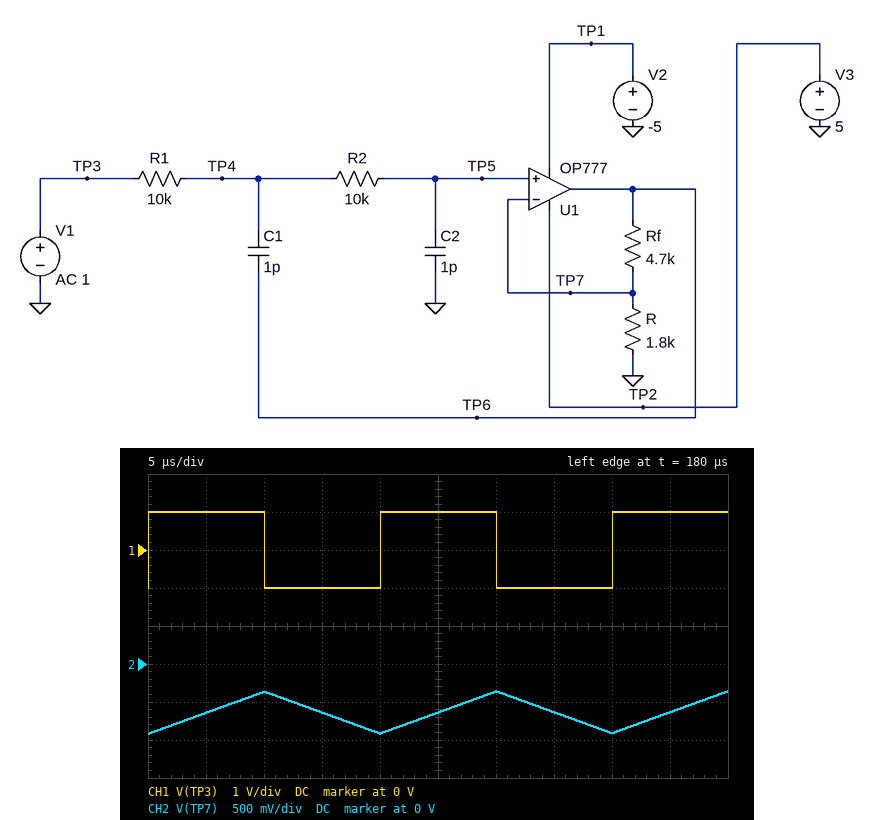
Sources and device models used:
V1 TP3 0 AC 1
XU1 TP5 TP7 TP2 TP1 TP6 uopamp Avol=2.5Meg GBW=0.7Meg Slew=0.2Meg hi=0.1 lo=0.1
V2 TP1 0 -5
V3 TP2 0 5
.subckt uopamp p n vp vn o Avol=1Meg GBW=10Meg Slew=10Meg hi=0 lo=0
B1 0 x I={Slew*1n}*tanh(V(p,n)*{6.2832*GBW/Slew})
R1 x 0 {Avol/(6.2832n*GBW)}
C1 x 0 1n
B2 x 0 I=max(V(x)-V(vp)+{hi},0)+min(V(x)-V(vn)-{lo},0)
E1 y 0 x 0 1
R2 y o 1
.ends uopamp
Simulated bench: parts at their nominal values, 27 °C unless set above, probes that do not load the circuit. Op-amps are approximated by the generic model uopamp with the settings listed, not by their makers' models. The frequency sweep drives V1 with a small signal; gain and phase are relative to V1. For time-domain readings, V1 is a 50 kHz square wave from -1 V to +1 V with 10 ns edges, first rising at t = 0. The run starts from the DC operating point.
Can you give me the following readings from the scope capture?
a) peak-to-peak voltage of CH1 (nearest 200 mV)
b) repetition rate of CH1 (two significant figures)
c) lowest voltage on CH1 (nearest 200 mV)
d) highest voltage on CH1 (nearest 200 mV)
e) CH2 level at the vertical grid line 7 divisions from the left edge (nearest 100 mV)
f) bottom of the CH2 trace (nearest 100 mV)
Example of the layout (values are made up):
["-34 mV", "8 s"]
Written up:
["2.0 V", "50 kHz", "-1.0 V", "1.0 V", "-600 mV", "-900 mV"]
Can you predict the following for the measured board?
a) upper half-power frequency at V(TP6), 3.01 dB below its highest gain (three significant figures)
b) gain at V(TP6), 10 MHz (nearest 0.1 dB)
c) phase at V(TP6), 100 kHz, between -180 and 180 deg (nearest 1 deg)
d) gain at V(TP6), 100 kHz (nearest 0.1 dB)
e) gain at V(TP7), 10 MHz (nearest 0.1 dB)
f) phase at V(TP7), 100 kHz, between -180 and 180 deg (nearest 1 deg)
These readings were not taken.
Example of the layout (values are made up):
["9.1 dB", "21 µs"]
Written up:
["203 kHz", "-29.0 dB", "-27 deg", "10.2 dB", "-40.1 dB", "-27 deg"]
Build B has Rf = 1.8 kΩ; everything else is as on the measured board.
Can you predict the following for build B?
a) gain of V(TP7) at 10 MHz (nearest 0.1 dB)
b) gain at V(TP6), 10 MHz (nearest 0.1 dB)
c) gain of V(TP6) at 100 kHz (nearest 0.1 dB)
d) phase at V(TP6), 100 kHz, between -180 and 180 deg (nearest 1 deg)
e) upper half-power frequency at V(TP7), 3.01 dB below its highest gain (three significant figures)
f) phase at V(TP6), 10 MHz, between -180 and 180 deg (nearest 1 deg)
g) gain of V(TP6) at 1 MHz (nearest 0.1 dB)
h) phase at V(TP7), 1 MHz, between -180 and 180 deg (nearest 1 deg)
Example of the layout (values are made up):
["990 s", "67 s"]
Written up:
["-35.0 dB", "-29.0 dB", "5.7 dB", "-16 deg", "366 kHz", "-161 deg", "-3.4 dB", "-81 deg"]
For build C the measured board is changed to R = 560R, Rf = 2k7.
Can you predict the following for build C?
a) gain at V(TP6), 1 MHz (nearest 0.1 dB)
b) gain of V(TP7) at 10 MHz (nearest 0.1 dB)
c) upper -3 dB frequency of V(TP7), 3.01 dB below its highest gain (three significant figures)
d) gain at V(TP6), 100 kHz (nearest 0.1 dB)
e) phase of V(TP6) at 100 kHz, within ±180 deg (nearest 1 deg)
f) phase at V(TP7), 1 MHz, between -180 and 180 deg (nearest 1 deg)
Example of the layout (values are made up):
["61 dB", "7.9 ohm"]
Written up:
["-2.9 dB", "-44.3 dB", "126 kHz", "13.2 dB", "-40 deg", "-94 deg"]
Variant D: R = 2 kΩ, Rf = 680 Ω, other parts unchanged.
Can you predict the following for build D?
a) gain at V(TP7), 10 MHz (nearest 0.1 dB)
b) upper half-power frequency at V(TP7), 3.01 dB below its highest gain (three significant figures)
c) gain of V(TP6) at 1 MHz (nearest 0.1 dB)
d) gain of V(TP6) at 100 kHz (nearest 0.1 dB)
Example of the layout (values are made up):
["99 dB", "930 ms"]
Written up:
["-31.5 dB", "544 kHz", "-3.9 dB", "2.4 dB"]
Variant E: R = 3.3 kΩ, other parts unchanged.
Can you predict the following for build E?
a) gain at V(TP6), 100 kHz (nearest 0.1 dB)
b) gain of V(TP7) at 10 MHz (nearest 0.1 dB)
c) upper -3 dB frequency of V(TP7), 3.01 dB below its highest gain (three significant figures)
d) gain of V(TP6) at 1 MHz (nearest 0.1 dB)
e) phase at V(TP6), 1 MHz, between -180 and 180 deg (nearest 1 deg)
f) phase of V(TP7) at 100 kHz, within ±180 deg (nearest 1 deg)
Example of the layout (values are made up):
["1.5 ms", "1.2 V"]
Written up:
["7.2 dB", "-36.7 dB", "302 kHz", "-3.2 dB", "-84 deg", "-19 deg"]
